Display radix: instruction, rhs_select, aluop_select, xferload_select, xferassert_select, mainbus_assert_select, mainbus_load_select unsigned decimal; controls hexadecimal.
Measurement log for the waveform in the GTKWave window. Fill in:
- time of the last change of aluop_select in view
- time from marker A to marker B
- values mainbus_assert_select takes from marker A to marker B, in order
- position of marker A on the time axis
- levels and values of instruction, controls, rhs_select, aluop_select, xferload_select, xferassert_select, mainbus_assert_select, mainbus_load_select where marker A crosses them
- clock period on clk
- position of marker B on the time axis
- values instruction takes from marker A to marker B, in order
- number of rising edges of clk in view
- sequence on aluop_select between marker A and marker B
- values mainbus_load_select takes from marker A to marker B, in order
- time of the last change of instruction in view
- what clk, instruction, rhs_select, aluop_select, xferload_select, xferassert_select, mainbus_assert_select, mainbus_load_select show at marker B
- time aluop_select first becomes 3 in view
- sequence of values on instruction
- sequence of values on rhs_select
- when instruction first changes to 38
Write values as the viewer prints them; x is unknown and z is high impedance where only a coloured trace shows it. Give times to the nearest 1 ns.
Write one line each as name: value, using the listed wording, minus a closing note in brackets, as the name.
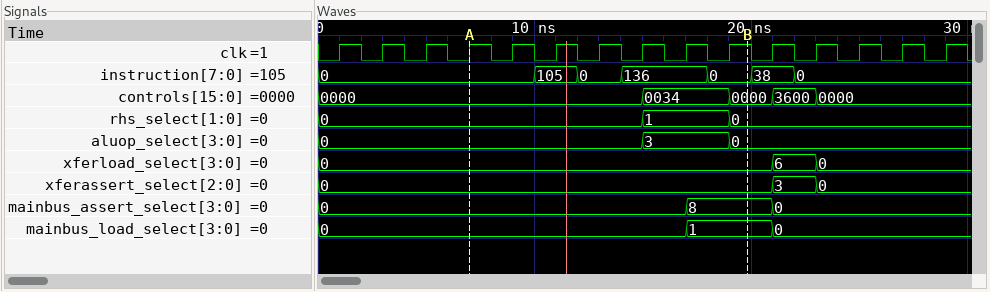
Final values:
time of the last change of aluop_select in view: 19 ns
time from marker A to marker B: 13 ns
values mainbus_assert_select takes from marker A to marker B, in order: 0, 8
position of marker A on the time axis: 7 ns
levels and values of instruction, controls, rhs_select, aluop_select, xferload_select, xferassert_select, mainbus_assert_select, mainbus_load_select where marker A crosses them: instruction=0, controls=0000, rhs_select=0, aluop_select=0, xferload_select=0, xferassert_select=0, mainbus_assert_select=0, mainbus_load_select=0
clock period on clk: 2 ns
position of marker B on the time axis: 20 ns
values instruction takes from marker A to marker B, in order: 0, 105, 0, 136, 0
number of rising edges of clk in view: 15
sequence on aluop_select between marker A and marker B: 0, 3, 0
values mainbus_load_select takes from marker A to marker B, in order: 0, 1
time of the last change of instruction in view: 22 ns
what clk, instruction, rhs_select, aluop_select, xferload_select, xferassert_select, mainbus_assert_select, mainbus_load_select show at marker B: clk=1, instruction=0, rhs_select=0, aluop_select=0, xferload_select=0, xferassert_select=0, mainbus_assert_select=8, mainbus_load_select=1
time aluop_select first becomes 3 in view: 15 ns
sequence of values on instruction: 0, 105, 0, 136, 0, 38, 0
sequence of values on rhs_select: 0, 1, 0
when instruction first changes to 38: 20 ns
